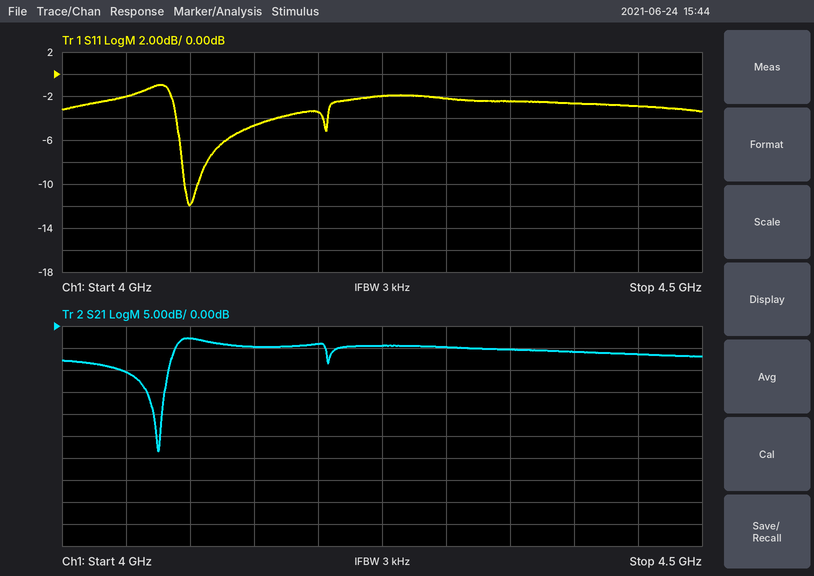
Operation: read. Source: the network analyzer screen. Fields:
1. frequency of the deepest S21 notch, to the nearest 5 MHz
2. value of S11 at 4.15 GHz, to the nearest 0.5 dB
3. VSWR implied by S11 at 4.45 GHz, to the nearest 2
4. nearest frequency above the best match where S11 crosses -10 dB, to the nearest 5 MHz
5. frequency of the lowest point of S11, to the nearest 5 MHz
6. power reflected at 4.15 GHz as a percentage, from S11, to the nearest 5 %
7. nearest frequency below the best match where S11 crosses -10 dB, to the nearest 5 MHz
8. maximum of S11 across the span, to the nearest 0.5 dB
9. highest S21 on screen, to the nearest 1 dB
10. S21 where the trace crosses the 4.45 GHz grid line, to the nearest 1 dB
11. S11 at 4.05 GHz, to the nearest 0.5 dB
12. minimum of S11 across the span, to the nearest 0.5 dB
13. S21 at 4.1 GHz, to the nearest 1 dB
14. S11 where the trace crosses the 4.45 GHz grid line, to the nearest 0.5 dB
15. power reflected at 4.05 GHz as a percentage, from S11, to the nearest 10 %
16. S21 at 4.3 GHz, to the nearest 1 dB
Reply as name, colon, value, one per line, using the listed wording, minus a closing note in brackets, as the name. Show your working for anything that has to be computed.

frequency of the deepest S21 notch, to the nearest 5 MHz: 4.075 GHz
value of S11 at 4.15 GHz, to the nearest 0.5 dB: -4.5 dB
VSWR implied by S11 at 4.45 GHz, to the nearest 2: |Γ| = 10^(-3/20) = 0.7079; VSWR = (1 + 0.7079)/(1 − 0.7079) ≈ 6
nearest frequency above the best match where S11 crosses -10 dB, to the nearest 5 MHz: 4.105 GHz
frequency of the lowest point of S11, to the nearest 5 MHz: 4.100 GHz
power reflected at 4.15 GHz as a percentage, from S11, to the nearest 5 %: 10^(-4.5/10) ≈ 35 %
nearest frequency below the best match where S11 crosses -10 dB, to the nearest 5 MHz: 4.095 GHz
maximum of S11 across the span, to the nearest 0.5 dB: -1.0 dB
highest S21 on screen, to the nearest 1 dB: -3 dB
S21 where the trace crosses the 4.45 GHz grid line, to the nearest 1 dB: -6 dB
S11 at 4.05 GHz, to the nearest 0.5 dB: -2.0 dB
minimum of S11 across the span, to the nearest 0.5 dB: -12.0 dB
S21 at 4.1 GHz, to the nearest 1 dB: -3 dB
S11 where the trace crosses the 4.45 GHz grid line, to the nearest 0.5 dB: -3.0 dB
power reflected at 4.05 GHz as a percentage, from S11, to the nearest 10 %: 10^(-2/10) ≈ 63.1 %, so 60 % to the nearest 10 %
S21 at 4.3 GHz, to the nearest 1 dB: -5 dB
